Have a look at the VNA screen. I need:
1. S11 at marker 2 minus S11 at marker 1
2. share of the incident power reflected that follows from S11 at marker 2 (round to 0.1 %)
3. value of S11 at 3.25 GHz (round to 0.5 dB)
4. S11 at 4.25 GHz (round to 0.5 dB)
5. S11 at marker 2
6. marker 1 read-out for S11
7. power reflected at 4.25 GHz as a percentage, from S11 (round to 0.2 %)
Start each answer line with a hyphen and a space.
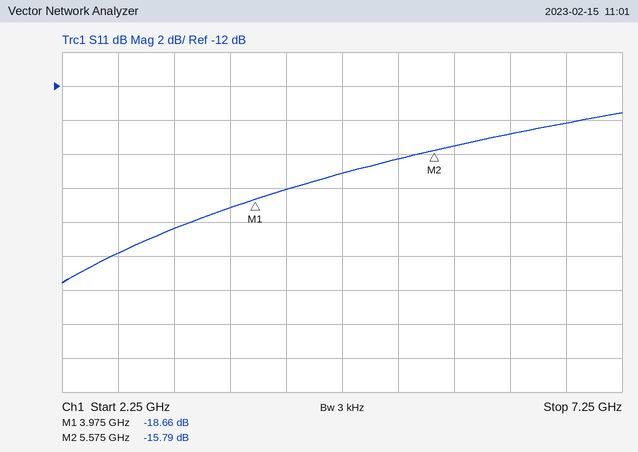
- 2.87 dB
- 2.6 %
- -20.5 dB
- -18.0 dB
- -15.79 dB
- -18.66 dB
- 1.6 %
